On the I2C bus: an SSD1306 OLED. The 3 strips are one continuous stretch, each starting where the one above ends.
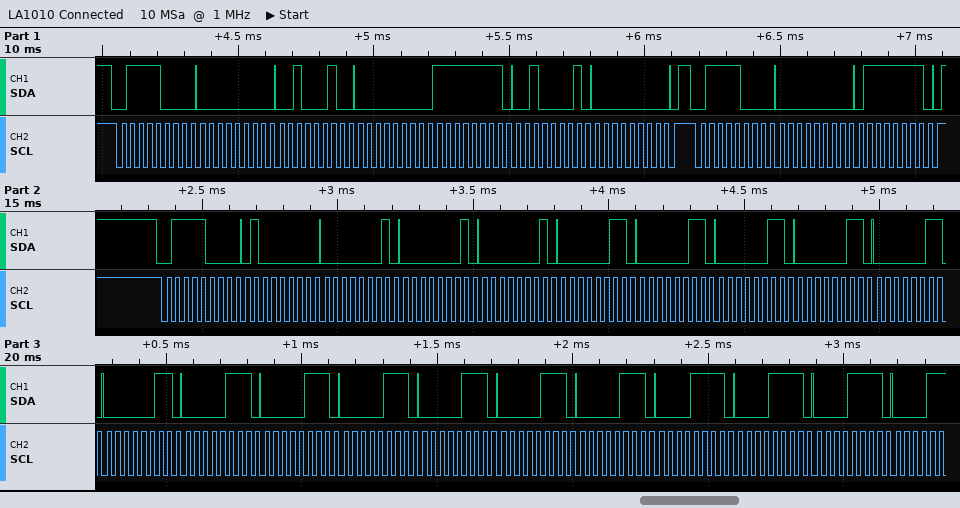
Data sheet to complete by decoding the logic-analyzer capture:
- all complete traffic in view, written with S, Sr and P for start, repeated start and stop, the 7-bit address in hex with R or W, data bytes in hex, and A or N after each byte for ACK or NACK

S 3CW A 00 A 22 A 00 A FF A 21 A 00 A P S 3CW A 00 A 7F A P S 3CW A 40 A 01 A 01 A 01 A 03 A 03 A 03 A 03 A 03 A 03 A 07 A 07 A 07 A 07 A 07 A 07 A 0F A 0F A 0F A
